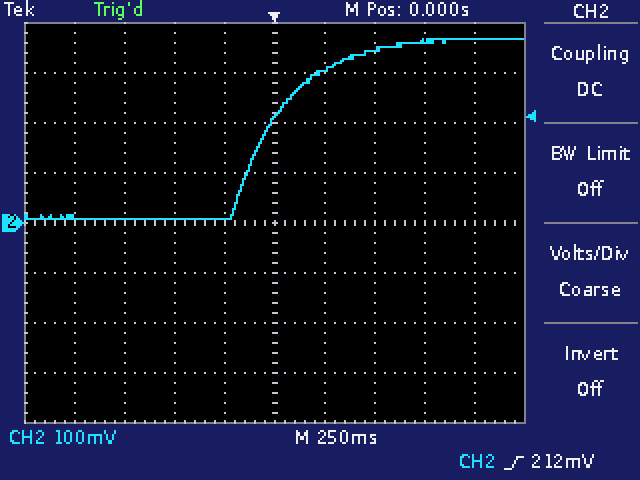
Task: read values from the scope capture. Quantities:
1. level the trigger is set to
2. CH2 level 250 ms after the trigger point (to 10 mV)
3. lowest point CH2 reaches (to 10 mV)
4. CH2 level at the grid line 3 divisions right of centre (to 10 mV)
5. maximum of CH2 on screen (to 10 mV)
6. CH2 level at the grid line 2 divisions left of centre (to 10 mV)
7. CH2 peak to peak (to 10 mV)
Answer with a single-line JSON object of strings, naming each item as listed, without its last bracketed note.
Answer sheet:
{"level the trigger is set to": "212 mV", "CH2 level 250 ms after the trigger point": "310 mV", "lowest point CH2 reaches": "10 mV", "CH2 level at the grid line 3 divisions right of centre": "360 mV", "maximum of CH2 on screen": "370 mV", "CH2 level at the grid line 2 divisions left of centre": "10 mV", "CH2 peak to peak": "360 mV"}
